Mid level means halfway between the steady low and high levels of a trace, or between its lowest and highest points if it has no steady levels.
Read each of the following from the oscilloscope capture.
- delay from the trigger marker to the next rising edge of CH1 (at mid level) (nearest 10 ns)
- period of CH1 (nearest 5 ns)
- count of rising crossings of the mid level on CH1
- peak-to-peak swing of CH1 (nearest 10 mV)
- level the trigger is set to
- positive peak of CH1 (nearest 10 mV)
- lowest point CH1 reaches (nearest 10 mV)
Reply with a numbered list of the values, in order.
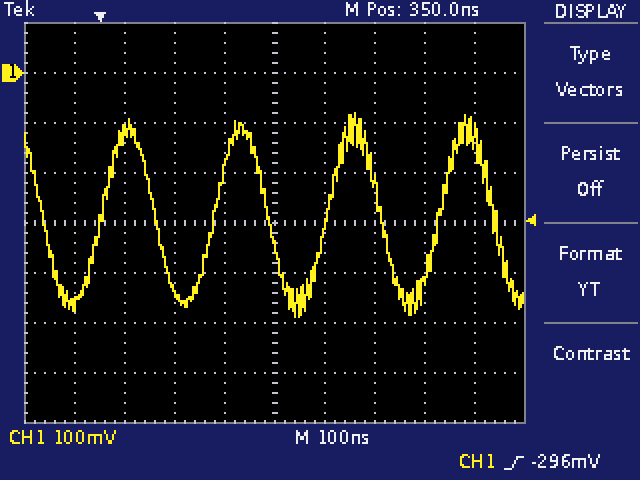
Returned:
1. 10 ns
2. 225 ns
3. 4
4. 410 mV
5. -296 mV
6. -80 mV
7. -490 mV
